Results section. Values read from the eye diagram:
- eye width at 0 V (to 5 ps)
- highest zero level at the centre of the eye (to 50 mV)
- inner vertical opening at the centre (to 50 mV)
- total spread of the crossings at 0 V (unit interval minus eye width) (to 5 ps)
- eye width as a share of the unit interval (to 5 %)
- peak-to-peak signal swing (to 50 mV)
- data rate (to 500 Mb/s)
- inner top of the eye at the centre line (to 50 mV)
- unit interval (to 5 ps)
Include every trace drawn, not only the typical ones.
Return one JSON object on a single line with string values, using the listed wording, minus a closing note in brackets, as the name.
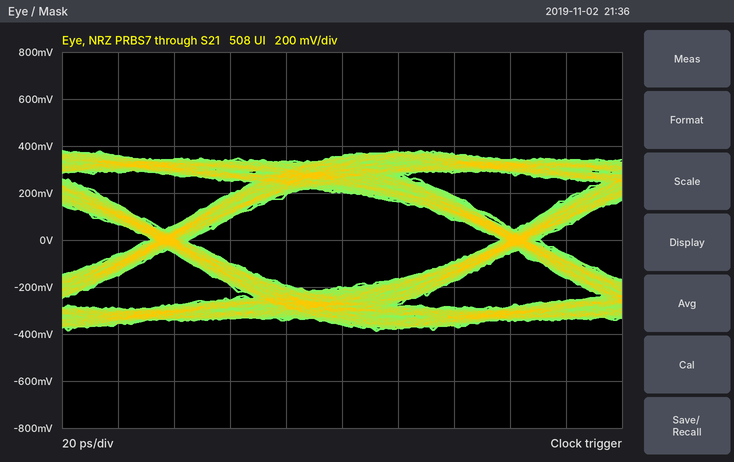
{"eye width at 0 V": "110 ps", "highest zero level at the centre of the eye": "-200 mV", "inner vertical opening at the centre": "400 mV", "total spread of the crossings at 0 V (unit interval minus eye width)": "15 ps", "eye width as a share of the unit interval": "90 %", "peak-to-peak signal swing": "750 mV", "data rate": "8.0 Gb/s", "inner top of the eye at the centre line": "200 mV", "unit interval": "125 ps"}
